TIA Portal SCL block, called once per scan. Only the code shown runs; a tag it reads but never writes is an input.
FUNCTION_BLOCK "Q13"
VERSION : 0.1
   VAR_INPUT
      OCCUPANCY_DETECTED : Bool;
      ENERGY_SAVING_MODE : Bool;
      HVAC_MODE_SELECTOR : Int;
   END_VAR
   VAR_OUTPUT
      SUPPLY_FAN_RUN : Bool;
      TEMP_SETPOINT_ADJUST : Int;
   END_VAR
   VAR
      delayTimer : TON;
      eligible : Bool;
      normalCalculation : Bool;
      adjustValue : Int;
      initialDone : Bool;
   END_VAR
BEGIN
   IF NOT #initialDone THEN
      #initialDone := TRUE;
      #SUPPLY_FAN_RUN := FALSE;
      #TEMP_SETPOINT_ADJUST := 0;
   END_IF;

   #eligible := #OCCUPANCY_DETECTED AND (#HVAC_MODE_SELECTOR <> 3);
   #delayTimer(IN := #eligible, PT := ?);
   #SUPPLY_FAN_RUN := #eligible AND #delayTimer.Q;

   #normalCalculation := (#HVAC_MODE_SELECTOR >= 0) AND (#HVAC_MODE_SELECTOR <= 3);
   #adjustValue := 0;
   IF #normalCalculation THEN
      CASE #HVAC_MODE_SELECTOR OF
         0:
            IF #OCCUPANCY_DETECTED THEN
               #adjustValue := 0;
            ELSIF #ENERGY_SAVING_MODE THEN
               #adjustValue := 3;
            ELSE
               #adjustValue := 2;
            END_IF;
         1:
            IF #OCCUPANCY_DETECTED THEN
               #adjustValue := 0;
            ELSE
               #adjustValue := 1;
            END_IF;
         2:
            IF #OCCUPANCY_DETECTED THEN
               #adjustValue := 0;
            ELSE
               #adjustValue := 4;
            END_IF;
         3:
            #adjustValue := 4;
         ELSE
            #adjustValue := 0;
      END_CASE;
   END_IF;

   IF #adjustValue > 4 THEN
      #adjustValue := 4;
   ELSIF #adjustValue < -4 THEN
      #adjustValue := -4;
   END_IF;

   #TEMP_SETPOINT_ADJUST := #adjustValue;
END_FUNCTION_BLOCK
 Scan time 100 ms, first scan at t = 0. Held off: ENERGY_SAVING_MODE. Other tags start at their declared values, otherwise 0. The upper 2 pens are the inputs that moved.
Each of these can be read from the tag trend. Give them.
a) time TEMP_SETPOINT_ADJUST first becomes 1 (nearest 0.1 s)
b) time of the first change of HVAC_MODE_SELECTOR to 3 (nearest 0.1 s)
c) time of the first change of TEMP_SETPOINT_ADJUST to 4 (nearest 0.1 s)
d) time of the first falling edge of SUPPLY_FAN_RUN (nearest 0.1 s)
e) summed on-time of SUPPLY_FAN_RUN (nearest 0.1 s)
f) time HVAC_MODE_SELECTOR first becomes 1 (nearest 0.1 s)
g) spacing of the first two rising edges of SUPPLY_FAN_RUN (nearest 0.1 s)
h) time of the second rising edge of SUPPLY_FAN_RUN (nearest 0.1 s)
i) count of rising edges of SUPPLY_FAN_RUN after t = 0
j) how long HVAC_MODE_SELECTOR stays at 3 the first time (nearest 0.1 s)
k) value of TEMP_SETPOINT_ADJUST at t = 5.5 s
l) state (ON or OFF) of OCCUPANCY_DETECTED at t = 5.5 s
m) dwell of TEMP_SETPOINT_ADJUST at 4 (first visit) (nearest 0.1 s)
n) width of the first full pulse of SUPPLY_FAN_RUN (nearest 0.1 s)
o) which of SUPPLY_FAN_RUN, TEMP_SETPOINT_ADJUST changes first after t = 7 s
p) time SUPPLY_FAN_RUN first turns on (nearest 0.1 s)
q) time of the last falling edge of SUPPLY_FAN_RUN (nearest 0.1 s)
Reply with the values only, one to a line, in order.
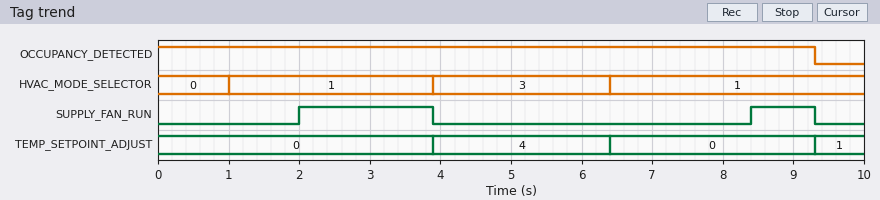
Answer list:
9.3 s
3.9 s
3.9 s
3.9 s
2.8 s
1.0 s
6.4 s
8.4 s
2
2.5 s
4
ON
2.5 s
1.9 s
SUPPLY_FAN_RUN
2.0 s
9.3 s
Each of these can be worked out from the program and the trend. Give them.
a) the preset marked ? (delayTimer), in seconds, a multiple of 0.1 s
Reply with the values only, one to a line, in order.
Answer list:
2.0 s
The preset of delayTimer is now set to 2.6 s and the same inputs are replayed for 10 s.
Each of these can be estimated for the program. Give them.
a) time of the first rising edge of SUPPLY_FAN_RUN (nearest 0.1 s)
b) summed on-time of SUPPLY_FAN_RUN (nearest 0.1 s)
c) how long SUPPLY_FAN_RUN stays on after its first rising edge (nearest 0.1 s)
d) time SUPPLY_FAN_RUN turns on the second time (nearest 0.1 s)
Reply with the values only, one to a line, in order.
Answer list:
2.6 s
1.6 s
1.3 s
9.0 s
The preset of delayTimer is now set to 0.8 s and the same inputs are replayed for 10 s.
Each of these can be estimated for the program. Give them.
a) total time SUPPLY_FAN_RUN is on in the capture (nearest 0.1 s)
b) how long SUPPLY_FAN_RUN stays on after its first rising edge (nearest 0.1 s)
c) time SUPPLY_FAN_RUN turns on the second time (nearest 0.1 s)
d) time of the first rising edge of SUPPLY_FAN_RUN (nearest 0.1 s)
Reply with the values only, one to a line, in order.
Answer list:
5.2 s
3.1 s
7.2 s
0.8 s
